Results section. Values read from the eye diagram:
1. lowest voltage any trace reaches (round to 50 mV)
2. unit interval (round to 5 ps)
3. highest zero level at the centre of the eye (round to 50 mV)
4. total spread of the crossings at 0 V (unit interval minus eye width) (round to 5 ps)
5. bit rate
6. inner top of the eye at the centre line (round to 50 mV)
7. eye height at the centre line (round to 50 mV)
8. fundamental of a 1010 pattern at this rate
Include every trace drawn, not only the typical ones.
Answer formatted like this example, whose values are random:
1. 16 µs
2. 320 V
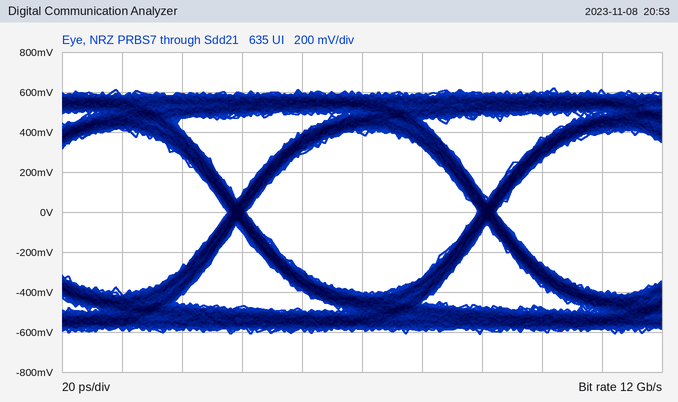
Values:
1. -600 mV
2. 85 ps
3. -400 mV
4. 5 ps
5. 12 Gb/s
6. 400 mV
7. 800 mV
8. 6 GHz
